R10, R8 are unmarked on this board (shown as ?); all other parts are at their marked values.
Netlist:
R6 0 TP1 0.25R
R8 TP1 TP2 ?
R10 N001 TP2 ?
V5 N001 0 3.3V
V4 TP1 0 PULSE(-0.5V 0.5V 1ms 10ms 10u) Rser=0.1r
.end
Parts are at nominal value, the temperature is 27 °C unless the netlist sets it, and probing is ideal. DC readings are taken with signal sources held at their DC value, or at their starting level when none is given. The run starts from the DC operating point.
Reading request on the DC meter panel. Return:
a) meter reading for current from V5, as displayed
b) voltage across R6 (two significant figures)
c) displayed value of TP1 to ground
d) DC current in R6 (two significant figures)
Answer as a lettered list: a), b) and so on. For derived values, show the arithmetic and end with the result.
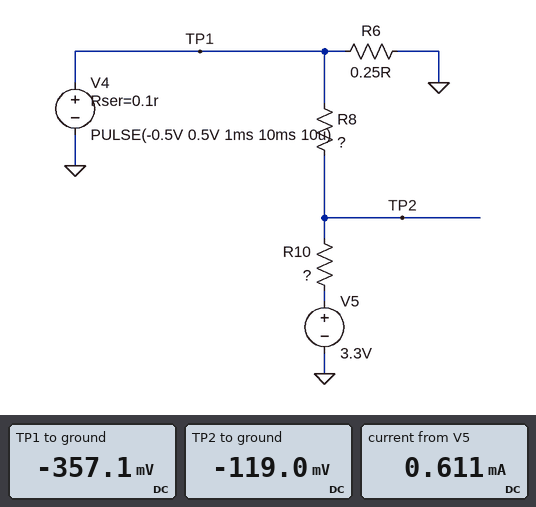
a) 0.611 mA
b) 0 V - (-357.1 mV) = 360 mV
c) -357.1 mV
d) (0 V - (-357.1 mV)) / 250 mΩ = 1.4 A
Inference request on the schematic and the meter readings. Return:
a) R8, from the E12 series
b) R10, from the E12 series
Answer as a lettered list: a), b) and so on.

a) 390 Ω
b) 5.6 kΩ
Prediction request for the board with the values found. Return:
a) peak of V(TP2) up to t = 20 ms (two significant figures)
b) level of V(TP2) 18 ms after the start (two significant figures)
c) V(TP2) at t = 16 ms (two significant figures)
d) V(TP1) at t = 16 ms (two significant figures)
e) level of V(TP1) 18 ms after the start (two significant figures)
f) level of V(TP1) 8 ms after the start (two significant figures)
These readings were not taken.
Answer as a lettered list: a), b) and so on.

a) 550 mV
b) 550 mV
c) 550 mV
d) 360 mV
e) 360 mV
f) 140 mV
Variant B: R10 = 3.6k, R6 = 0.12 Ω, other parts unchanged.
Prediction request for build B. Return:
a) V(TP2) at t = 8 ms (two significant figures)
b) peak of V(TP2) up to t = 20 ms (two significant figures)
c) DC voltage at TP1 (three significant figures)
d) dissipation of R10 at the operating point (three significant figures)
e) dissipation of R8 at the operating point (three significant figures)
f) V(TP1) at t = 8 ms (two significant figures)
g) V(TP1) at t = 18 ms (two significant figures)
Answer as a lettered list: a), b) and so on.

a) 420 mV
b) 570 mV
c) -273 mV
d) 2.89 mW
e) 313 µW
f) 110 mV
g) 270 mV
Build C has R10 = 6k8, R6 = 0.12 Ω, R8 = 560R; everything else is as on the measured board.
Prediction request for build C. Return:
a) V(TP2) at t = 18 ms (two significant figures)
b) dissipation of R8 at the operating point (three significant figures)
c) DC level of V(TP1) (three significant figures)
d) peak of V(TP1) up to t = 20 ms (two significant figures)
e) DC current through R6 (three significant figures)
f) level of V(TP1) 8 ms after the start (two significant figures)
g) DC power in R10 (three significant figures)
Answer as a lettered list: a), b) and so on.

a) 500 mV
b) 132 µW
c) -273 mV
d) 270 mV
e) 2.27 A
f) 110 mV
g) 1.60 mW
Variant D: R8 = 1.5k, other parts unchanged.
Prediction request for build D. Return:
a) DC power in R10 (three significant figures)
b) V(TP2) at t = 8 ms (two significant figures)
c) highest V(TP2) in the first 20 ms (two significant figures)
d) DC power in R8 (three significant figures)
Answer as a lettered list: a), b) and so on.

a) 1.49 mW
b) 810 mV
c) 980 mV
d) 398 µW
